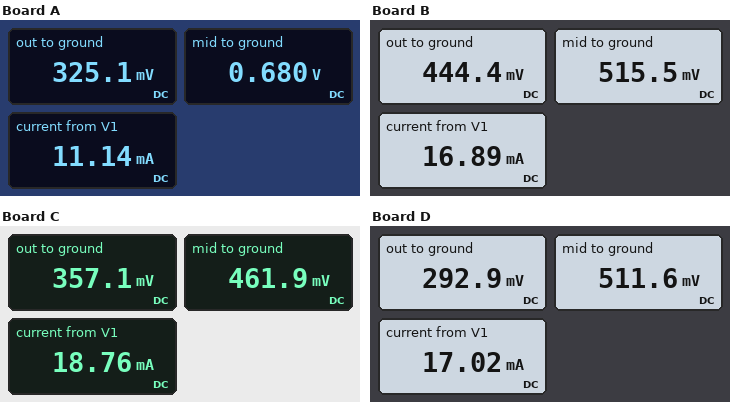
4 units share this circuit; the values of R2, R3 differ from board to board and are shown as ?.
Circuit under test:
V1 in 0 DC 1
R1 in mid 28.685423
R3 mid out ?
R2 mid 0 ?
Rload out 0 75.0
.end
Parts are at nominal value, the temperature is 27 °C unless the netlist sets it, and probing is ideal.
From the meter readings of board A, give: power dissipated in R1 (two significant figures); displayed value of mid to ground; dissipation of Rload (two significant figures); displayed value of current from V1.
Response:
3.6 mW
0.680 V
1.4 mW
11.14 mA
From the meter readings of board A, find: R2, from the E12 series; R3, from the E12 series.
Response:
100 Ω
82 Ω
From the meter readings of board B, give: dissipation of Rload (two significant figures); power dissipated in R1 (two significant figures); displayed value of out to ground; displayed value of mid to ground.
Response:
2.6 mW
8.2 mW
444.4 mV
515.5 mV
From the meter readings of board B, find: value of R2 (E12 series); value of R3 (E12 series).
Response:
47 Ω
12 Ω
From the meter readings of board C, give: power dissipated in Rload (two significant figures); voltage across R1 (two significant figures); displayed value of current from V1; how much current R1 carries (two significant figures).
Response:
1.7 mW
540 mV
18.76 mA
19 mA
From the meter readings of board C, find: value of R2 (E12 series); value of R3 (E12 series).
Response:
33 Ω
22 Ω
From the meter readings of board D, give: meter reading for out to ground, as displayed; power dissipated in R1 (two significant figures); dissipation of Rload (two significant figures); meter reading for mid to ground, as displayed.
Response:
292.9 mV
8.3 mW
1.1 mW
511.6 mV
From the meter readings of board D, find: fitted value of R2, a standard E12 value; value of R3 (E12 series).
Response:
39 Ω
56 Ω
